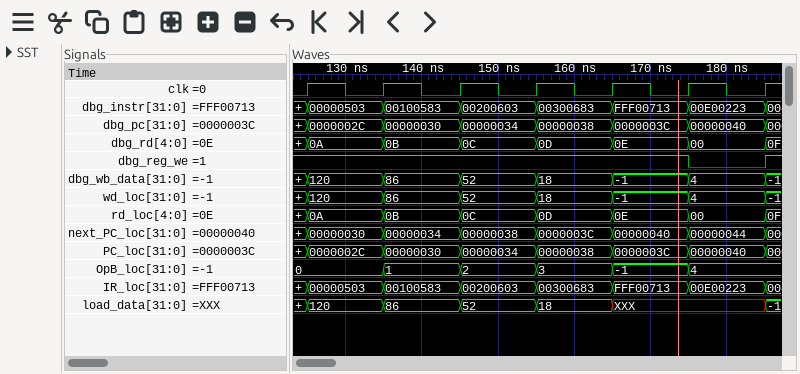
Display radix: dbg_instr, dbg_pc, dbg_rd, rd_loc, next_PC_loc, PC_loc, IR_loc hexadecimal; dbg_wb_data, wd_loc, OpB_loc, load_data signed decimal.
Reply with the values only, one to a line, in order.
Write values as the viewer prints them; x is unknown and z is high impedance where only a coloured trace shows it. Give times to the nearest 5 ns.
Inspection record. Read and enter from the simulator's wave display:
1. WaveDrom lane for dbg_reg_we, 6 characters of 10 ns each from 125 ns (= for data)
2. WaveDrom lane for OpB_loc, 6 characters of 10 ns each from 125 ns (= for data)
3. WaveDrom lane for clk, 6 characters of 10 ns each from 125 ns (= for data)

{name: 'dbg_reg_we', wave: '1....0'}
{name: 'OpB_loc', wave: '======', data: '0 1 2 3 -1 4'}
{name: 'clk', wave: 'p.....'}
